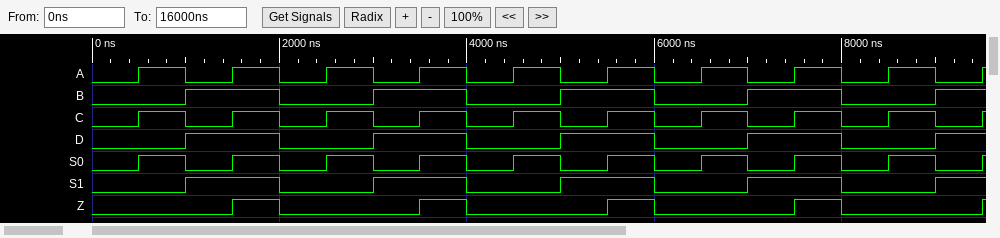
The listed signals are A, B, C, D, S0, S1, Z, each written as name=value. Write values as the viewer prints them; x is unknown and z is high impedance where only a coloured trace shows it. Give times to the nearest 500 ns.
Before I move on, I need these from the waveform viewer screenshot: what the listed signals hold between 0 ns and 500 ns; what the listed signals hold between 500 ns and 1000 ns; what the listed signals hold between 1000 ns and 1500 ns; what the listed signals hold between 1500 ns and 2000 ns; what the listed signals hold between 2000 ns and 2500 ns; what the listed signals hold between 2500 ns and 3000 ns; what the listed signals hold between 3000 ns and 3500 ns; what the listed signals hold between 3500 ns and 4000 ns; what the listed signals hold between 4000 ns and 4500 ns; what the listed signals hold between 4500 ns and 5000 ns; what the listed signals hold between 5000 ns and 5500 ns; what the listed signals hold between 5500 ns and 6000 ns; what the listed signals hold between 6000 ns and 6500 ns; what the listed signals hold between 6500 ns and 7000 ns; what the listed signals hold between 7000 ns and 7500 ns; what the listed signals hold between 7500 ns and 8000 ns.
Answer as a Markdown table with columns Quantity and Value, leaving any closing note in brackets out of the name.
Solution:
| Quantity | Value |
|---|---|
| what the listed signals hold between 0 ns and 500 ns | A=0, B=0, C=0, D=0, S0=0, S1=0, Z=0 |
| what the listed signals hold between 500 ns and 1000 ns | A=1, B=0, C=1, D=0, S0=1, S1=0, Z=0 |
| what the listed signals hold between 1000 ns and 1500 ns | A=0, B=1, C=0, D=1, S0=0, S1=1, Z=0 |
| what the listed signals hold between 1500 ns and 2000 ns | A=1, B=1, C=1, D=1, S0=1, S1=1, Z=1 |
| what the listed signals hold between 2000 ns and 2500 ns | A=0, B=0, C=0, D=0, S0=0, S1=0, Z=0 |
| what the listed signals hold between 2500 ns and 3000 ns | A=1, B=0, C=1, D=0, S0=1, S1=0, Z=0 |
| what the listed signals hold between 3000 ns and 3500 ns | A=0, B=1, C=0, D=1, S0=0, S1=1, Z=0 |
| what the listed signals hold between 3500 ns and 4000 ns | A=1, B=1, C=1, D=1, S0=1, S1=1, Z=1 |
| what the listed signals hold between 4000 ns and 4500 ns | A=0, B=0, C=0, D=0, S0=0, S1=0, Z=0 |
| what the listed signals hold between 4500 ns and 5000 ns | A=1, B=0, C=1, D=0, S0=1, S1=0, Z=0 |
| what the listed signals hold between 5000 ns and 5500 ns | A=0, B=1, C=0, D=1, S0=0, S1=1, Z=0 |
| what the listed signals hold between 5500 ns and 6000 ns | A=1, B=1, C=1, D=1, S0=1, S1=1, Z=1 |
| what the listed signals hold between 6000 ns and 6500 ns | A=0, B=0, C=0, D=0, S0=0, S1=0, Z=0 |
| what the listed signals hold between 6500 ns and 7000 ns | A=1, B=0, C=1, D=0, S0=1, S1=0, Z=0 |
| what the listed signals hold between 7000 ns and 7500 ns | A=0, B=1, C=0, D=1, S0=0, S1=1, Z=0 |
| what the listed signals hold between 7500 ns and 8000 ns | A=1, B=1, C=1, D=1, S0=1, S1=1, Z=1 |
